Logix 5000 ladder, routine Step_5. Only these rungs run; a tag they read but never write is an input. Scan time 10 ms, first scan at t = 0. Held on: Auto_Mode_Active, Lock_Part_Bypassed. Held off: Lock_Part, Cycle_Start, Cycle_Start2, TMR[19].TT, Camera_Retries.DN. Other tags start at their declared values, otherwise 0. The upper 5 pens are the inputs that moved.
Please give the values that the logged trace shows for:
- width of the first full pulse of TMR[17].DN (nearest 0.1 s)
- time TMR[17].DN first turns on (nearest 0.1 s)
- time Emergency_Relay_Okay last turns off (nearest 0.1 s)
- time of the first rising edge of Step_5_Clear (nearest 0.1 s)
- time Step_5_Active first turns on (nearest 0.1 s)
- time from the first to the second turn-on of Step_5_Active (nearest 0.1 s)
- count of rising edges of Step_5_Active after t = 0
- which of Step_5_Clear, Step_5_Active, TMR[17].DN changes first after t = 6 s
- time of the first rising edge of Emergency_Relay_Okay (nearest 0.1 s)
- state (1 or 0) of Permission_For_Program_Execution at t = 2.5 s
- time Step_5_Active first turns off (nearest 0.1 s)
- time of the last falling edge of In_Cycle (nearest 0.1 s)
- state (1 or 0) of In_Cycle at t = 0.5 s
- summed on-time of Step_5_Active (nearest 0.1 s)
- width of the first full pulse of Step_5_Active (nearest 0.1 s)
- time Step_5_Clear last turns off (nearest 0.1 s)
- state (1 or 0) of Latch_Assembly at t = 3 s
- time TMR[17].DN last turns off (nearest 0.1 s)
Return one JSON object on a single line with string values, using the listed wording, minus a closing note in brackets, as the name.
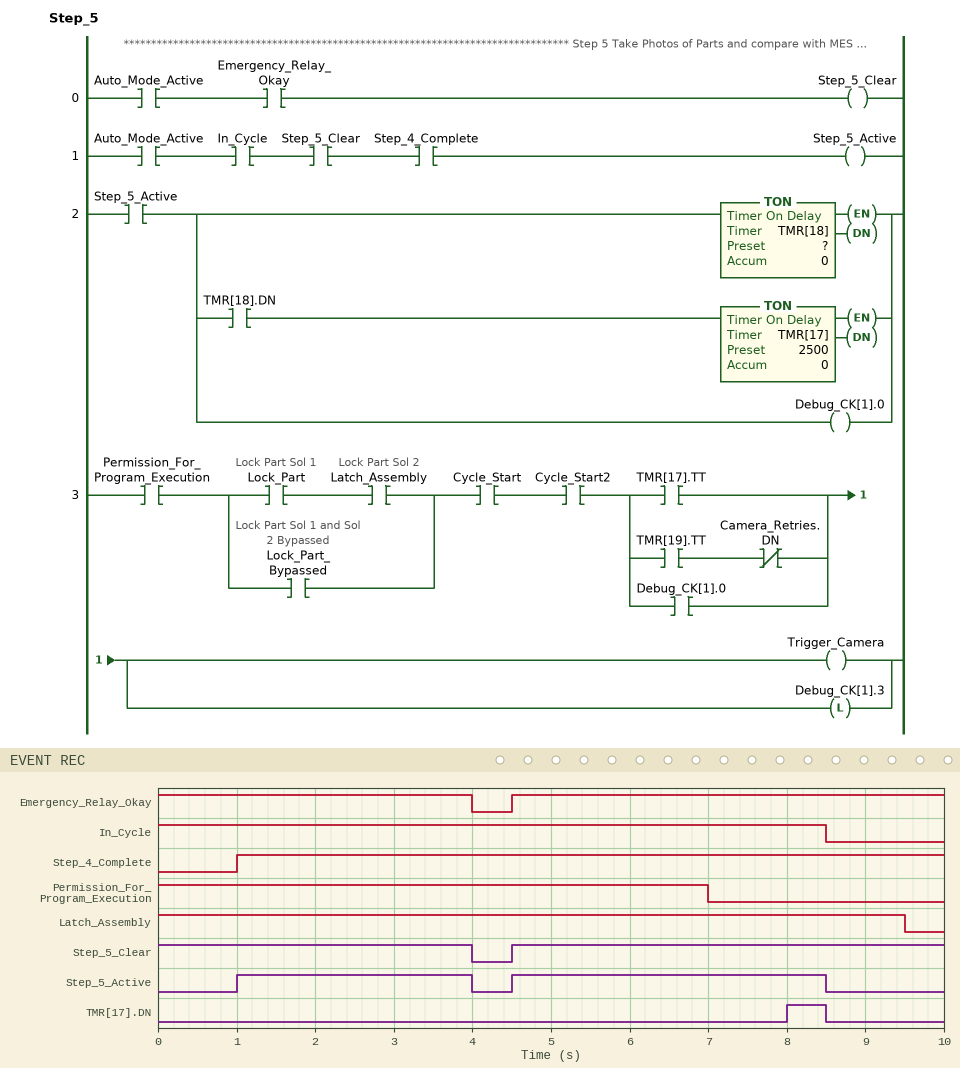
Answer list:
{"width of the first full pulse of TMR[17].DN": "0.5 s", "time TMR[17].DN first turns on": "8.0 s", "time Emergency_Relay_Okay last turns off": "4.0 s", "time of the first rising edge of Step_5_Clear": "4.5 s", "time Step_5_Active first turns on": "1.0 s", "time from the first to the second turn-on of Step_5_Active": "3.5 s", "count of rising edges of Step_5_Active after t = 0": "2", "which of Step_5_Clear, Step_5_Active, TMR[17].DN changes first after t = 6 s": "TMR[17].DN", "time of the first rising edge of Emergency_Relay_Okay": "4.5 s", "state (1 or 0) of Permission_For_Program_Execution at t = 2.5 s": "1", "time Step_5_Active first turns off": "4.0 s", "time of the last falling edge of In_Cycle": "8.5 s", "state (1 or 0) of In_Cycle at t = 0.5 s": "1", "summed on-time of Step_5_Active": "7.0 s", "width of the first full pulse of Step_5_Active": "3.0 s", "time Step_5_Clear last turns off": "4.0 s", "state (1 or 0) of Latch_Assembly at t = 3 s": "1", "time TMR[17].DN last turns off": "8.5 s"}
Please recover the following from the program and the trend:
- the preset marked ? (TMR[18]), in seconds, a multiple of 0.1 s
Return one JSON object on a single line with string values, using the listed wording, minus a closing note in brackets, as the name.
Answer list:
{"the preset marked ? (TMR[18]), in seconds, a multiple of 0.1 s": "1.0 s"}
